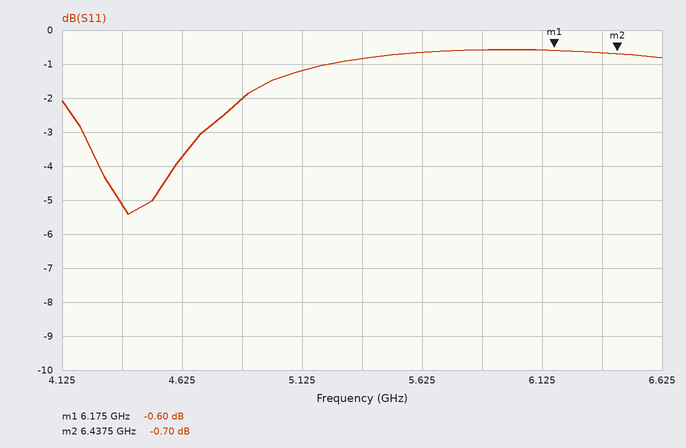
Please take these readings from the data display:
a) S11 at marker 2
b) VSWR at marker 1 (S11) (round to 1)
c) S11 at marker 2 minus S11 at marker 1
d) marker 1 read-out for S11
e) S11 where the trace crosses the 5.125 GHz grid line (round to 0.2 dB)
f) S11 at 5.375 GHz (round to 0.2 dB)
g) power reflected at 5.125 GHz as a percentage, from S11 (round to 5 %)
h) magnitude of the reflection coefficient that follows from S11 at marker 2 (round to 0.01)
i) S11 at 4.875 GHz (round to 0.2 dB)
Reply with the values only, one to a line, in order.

-0.70 dB
29
-0.10 dB
-0.60 dB
-1.2 dB
-0.8 dB
75 %
0.92
-2.0 dB
